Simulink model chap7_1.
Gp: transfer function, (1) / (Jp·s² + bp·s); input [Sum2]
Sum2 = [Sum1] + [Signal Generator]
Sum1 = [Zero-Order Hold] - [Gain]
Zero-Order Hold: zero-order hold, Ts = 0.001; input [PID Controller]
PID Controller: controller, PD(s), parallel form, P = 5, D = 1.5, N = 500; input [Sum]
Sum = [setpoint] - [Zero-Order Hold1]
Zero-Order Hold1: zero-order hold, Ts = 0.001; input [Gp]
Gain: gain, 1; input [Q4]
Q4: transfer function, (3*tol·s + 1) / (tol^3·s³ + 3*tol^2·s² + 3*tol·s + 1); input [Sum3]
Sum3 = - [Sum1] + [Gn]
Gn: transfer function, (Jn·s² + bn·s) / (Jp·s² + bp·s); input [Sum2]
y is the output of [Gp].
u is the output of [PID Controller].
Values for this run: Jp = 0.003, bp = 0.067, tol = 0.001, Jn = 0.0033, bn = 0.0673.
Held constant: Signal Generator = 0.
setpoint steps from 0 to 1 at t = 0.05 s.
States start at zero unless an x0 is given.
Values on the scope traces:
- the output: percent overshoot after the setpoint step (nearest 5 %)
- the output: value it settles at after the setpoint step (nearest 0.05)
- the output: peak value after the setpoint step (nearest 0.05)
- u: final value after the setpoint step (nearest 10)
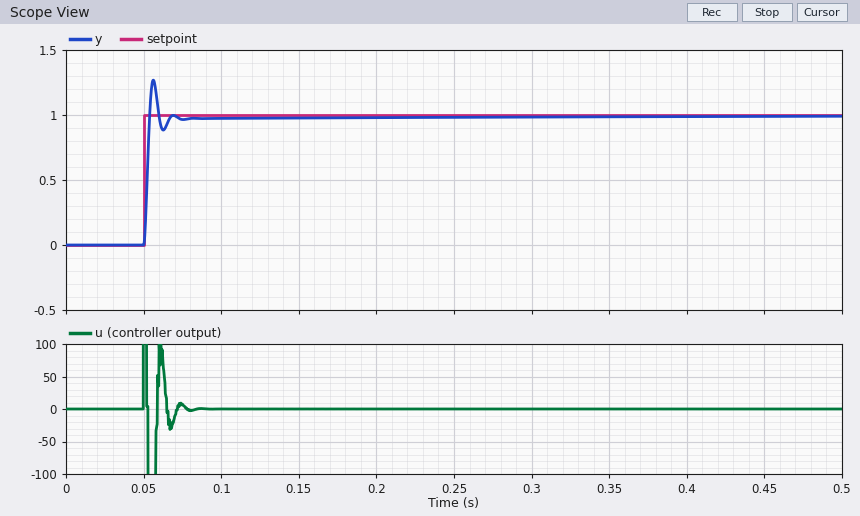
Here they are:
25 %
1.00
1.25
0
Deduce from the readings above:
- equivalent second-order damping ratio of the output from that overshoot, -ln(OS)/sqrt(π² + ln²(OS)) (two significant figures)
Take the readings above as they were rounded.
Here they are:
0.40
